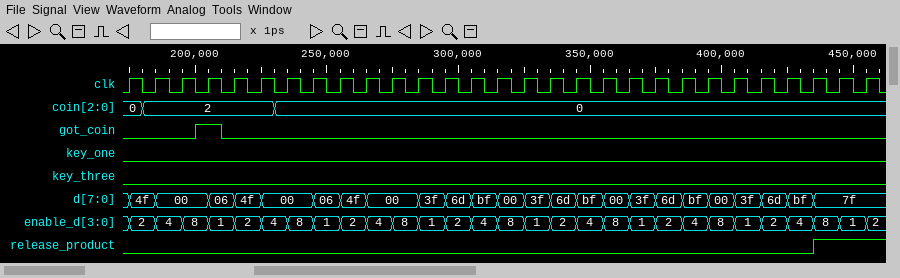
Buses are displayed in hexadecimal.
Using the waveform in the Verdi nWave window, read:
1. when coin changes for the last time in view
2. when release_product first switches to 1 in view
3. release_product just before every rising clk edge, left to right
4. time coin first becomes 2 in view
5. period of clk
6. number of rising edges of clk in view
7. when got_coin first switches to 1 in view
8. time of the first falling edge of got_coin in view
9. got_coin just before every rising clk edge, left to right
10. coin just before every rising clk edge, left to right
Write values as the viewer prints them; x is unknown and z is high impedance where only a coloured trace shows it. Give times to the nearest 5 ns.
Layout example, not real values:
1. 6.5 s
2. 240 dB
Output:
1. 230 ns
2. 435 ns
3. 0 0 0 0 0 0 0 0 0 0 0 0 0 0 0 0 0 0 0 0 0 0 0 0 0 0 0 1 1
4. 180 ns
5. 10 ns
6. 29
7. 200 ns
8. 210 ns
9. 0 0 0 1 0 0 0 0 0 0 0 0 0 0 0 0 0 0 0 0 0 0 0 0 0 0 0 0 0
10. 0, 2, 2, 2, 2, 2, 0, 0, 0, 0, 0, 0, 0, 0, 0, 0, 0, 0, 0, 0, 0, 0, 0, 0, 0, 0, 0, 0, 0
